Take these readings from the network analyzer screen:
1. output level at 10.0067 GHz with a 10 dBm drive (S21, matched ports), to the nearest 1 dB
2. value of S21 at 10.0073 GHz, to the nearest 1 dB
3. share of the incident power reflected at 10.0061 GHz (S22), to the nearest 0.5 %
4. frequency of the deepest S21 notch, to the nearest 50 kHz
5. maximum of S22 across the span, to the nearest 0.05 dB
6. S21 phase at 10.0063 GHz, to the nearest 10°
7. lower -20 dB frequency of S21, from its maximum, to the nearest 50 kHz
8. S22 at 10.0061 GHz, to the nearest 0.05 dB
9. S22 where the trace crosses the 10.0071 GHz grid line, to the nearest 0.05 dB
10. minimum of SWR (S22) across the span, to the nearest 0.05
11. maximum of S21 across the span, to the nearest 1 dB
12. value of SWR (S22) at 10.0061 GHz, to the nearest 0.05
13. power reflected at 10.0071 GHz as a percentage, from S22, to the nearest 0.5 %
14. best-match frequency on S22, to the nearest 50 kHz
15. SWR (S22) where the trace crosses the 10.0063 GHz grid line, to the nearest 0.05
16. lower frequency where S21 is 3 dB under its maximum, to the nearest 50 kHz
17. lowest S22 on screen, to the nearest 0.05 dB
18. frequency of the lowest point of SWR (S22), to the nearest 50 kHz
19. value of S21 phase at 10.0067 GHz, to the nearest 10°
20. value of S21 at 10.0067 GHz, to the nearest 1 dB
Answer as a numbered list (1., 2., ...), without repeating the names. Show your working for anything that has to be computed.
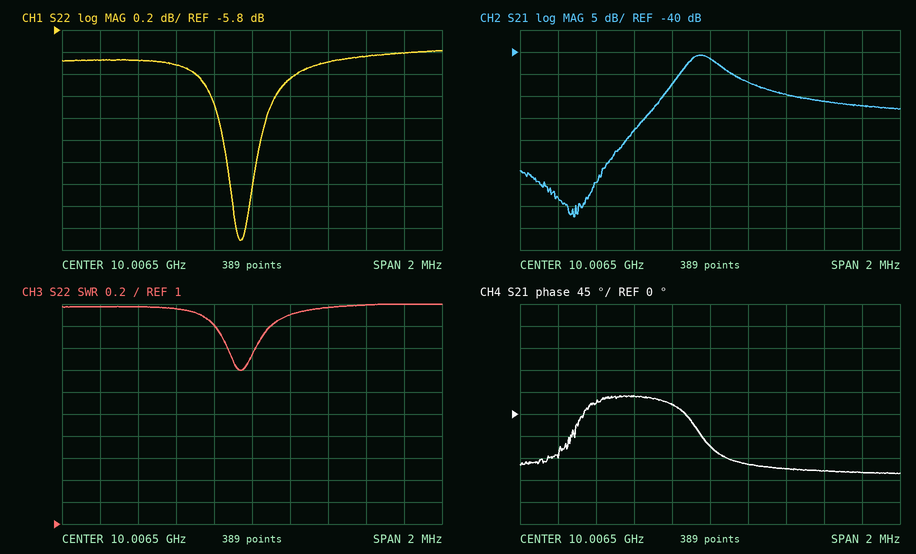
1. 10 dBm + (-47 dB) = -37 dBm
2. -52 dB
3. 10^(-6.1/10) ≈ 24.5 %
4. 10.00580 GHz
5. -6.00 dB
6. 20°
7. 10.00605 GHz
8. -6.10 dB
9. -6.05 dB
10. 2.40
11. -41 dB
12. 2.95
13. 10^(-6.05/10) ≈ 24.8 %, so 25.0 % to the nearest 0.5 %
14. 10.00645 GHz
15. 2.80
16. 10.00635 GHz
17. -7.70 dB
18. 10.00645 GHz
19. -100°
20. -47 dB
